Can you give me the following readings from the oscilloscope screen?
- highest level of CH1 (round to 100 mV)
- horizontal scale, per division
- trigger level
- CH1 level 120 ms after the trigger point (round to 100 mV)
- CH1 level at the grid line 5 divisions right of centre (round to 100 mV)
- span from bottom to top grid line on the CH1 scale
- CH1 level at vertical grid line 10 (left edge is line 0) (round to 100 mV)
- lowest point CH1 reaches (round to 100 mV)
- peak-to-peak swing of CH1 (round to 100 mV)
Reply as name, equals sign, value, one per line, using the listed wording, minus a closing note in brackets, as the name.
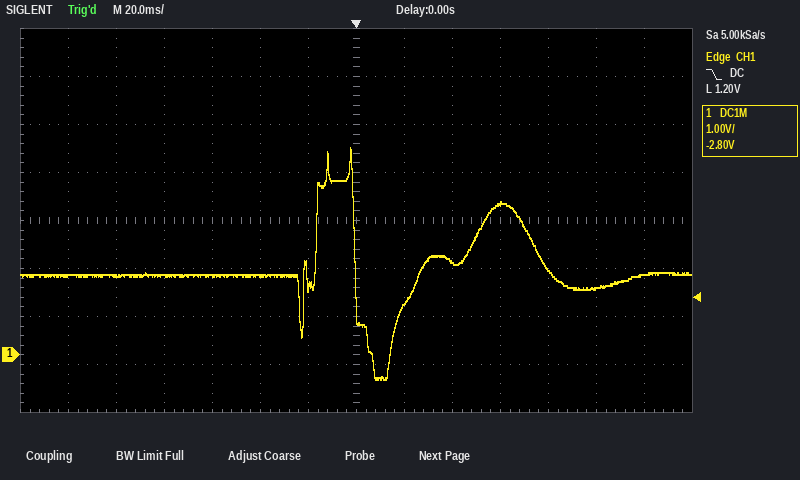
highest level of CH1 = 4.3 V
horizontal scale, per division = 20 ms
trigger level = 1.20 V
CH1 level 120 ms after the trigger point = 1.7 V
CH1 level at the grid line 5 divisions right of centre = 1.4 V
span from bottom to top grid line on the CH1 scale = 8 V
CH1 level at vertical grid line 10 (left edge is line 0) = 3.2 V
lowest point CH1 reaches = -500 mV
peak-to-peak swing of CH1 = 4.8 V
